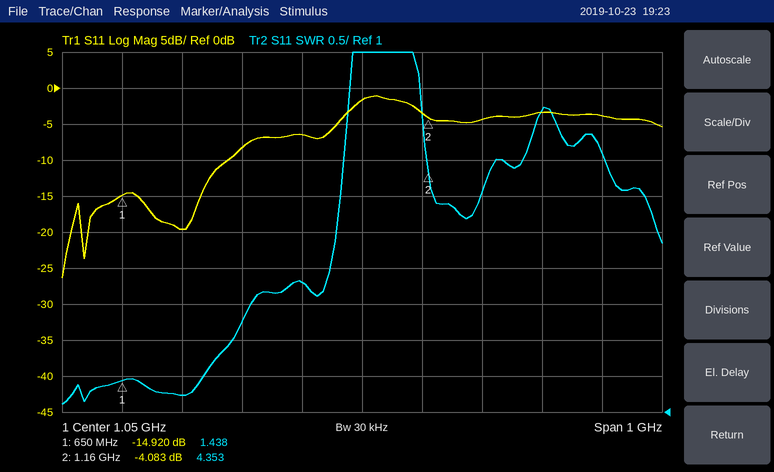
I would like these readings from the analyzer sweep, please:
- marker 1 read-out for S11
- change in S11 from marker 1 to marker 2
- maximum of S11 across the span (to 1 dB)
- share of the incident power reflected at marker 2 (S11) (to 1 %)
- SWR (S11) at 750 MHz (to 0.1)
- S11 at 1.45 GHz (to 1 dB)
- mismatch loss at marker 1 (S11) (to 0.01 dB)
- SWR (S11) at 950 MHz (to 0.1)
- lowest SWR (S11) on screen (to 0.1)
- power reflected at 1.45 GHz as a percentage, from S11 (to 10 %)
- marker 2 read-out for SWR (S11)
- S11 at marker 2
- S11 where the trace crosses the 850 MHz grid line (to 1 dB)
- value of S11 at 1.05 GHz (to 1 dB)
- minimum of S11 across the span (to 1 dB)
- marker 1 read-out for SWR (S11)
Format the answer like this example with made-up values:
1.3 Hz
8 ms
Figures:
-14.920 dB
10.837 dB
-1 dB
39 %
1.2
-4 dB
0.14 dB
2.8
1.1
40 %
4.353
-4.083 dB
-8 dB
-2 dB
-26 dB
1.438
